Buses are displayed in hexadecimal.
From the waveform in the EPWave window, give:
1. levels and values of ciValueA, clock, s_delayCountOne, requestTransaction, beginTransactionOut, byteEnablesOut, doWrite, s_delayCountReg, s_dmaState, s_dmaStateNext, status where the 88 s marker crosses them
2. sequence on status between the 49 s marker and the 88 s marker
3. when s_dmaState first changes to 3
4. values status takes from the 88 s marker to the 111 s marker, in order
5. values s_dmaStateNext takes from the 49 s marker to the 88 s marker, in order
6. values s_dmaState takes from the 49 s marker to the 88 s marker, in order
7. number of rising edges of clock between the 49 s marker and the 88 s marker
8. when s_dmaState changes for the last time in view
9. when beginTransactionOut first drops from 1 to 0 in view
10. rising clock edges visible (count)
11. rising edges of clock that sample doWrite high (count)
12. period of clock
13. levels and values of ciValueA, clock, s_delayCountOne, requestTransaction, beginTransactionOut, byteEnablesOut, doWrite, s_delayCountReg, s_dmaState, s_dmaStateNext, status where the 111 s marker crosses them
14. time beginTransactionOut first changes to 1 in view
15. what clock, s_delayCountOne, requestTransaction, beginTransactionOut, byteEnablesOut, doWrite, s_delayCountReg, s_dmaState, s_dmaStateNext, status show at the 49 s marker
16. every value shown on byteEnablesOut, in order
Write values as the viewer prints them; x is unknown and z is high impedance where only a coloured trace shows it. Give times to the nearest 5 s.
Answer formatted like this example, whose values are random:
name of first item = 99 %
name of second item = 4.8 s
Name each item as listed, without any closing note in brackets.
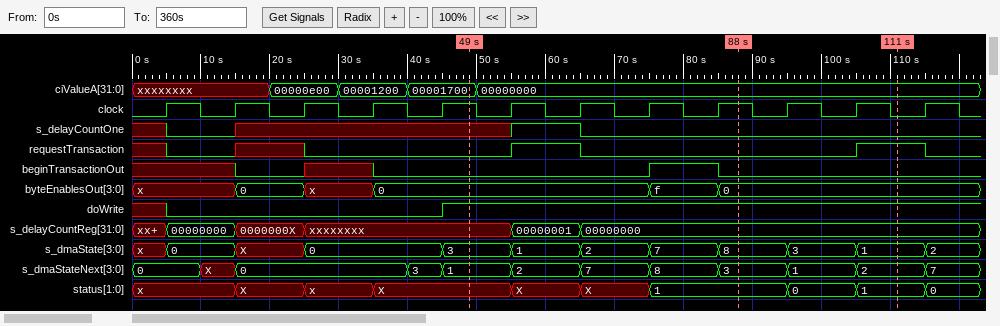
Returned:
levels and values of ciValueA, clock, s_delayCountOne, requestTransaction, beginTransactionOut, byteEnablesOut, doWrite, s_delayCountReg, s_dmaState, s_dmaStateNext, status where the 88 s marker crosses them = ciValueA=00000000, clock=1, s_delayCountOne=0, requestTransaction=0, beginTransactionOut=0, byteEnablesOut=0, doWrite=1, s_delayCountReg=00000000, s_dmaState=8, s_dmaStateNext=3, status=1
sequence on status between the 49 s marker and the 88 s marker = X, X, X, 1
when s_dmaState first changes to 3 = 45 s
values status takes from the 88 s marker to the 111 s marker, in order = 1, 0, 1
values s_dmaStateNext takes from the 49 s marker to the 88 s marker, in order = 1, 2, 7, 8, 3
values s_dmaState takes from the 49 s marker to the 88 s marker, in order = 3, 1, 2, 7, 8
number of rising edges of clock between the 49 s marker and the 88 s marker = 4
when s_dmaState changes for the last time in view = 115 s
when beginTransactionOut first drops from 1 to 0 in view = 85 s
rising clock edges visible = 12
rising edges of clock that sample doWrite high = 7
period of clock = 10 s
levels and values of ciValueA, clock, s_delayCountOne, requestTransaction, beginTransactionOut, byteEnablesOut, doWrite, s_delayCountReg, s_dmaState, s_dmaStateNext, status where the 111 s marker crosses them = ciValueA=00000000, clock=0, s_delayCountOne=0, requestTransaction=1, beginTransactionOut=0, byteEnablesOut=0, doWrite=1, s_delayCountReg=00000000, s_dmaState=1, s_dmaStateNext=2, status=1
time beginTransactionOut first changes to 1 in view = 75 s
what clock, s_delayCountOne, requestTransaction, beginTransactionOut, byteEnablesOut, doWrite, s_delayCountReg, s_dmaState, s_dmaStateNext, status show at the 49 s marker = clock=1, s_delayCountOne=x, requestTransaction=0, beginTransactionOut=0, byteEnablesOut=0, doWrite=1, s_delayCountReg=xxxxxxxx, s_dmaState=3, s_dmaStateNext=1, status=X
every value shown on byteEnablesOut, in order = x, 0, x, 0, f, 0
